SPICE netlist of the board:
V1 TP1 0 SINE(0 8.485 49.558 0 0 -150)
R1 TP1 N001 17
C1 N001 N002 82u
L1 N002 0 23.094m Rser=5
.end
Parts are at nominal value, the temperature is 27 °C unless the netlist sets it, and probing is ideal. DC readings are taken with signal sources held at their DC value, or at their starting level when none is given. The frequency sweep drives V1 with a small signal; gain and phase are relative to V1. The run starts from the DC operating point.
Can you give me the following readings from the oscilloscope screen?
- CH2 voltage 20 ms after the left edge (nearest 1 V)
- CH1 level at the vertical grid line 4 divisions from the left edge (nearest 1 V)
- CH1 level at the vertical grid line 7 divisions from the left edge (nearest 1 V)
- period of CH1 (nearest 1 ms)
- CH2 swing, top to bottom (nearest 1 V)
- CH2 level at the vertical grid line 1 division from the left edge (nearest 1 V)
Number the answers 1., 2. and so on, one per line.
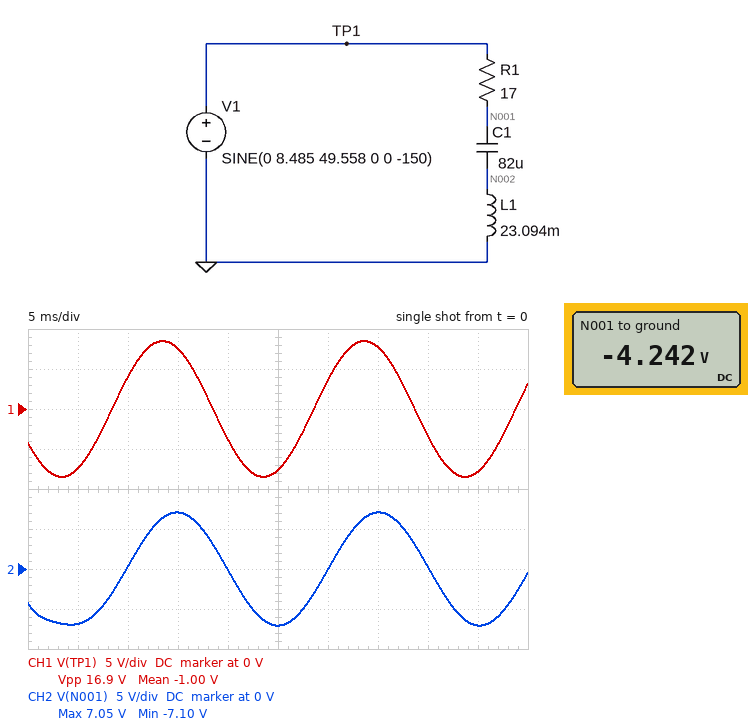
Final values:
1. 0 V
2. -4 V
3. 8 V
4. 20 ms
5. 14 V
6. -7 V
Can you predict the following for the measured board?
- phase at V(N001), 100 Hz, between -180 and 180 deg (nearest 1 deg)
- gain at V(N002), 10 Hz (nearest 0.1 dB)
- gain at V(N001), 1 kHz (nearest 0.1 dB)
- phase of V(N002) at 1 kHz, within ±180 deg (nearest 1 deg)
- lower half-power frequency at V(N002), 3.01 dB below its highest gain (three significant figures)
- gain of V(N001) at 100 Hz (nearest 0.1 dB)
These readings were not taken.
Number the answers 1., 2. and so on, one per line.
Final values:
1. -32 deg
2. -31.4 dB
3. -0.1 dB
4. 7 deg
5. 105 Hz
6. -10.2 dB
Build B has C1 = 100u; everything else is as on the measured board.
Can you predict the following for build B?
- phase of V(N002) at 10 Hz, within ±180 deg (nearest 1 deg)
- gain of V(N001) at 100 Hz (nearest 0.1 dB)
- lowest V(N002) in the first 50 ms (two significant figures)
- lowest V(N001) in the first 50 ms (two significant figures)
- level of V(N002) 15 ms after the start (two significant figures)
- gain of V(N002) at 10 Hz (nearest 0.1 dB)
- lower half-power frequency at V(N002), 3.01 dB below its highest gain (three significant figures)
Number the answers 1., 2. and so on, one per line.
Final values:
1. 98 deg
2. -12.6 dB
3. -2.2 V
4. -6.7 V
5. -1.5 V
6. -29.7 dB
7. 102 Hz
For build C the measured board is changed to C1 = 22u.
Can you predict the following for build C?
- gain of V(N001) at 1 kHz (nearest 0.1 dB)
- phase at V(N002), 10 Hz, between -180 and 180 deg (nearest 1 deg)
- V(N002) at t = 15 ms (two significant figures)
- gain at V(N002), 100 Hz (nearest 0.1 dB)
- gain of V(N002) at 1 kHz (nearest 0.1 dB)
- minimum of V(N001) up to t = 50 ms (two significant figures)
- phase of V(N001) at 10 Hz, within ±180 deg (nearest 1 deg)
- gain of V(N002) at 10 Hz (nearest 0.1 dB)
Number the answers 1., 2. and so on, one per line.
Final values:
1. -0.1 dB
2. 104 deg
3. -510 mV
4. -12.1 dB
5. 0.3 dB
6. -8.4 V
7. -1 deg
8. -42.8 dB
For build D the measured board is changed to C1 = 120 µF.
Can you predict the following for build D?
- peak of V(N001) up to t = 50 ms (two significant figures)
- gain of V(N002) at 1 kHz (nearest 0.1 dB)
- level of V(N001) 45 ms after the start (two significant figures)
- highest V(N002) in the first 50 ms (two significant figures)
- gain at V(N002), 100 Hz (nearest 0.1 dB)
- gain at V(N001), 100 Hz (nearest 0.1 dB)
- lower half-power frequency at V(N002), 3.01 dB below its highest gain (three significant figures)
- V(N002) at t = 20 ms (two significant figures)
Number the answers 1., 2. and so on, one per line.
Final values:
1. 5.8 V
2. 0 dB
3. -5.7 V
4. 2.5 V
5. -3.1 dB
6. -12.6 dB
7. 102 Hz
8. -2.1 V
